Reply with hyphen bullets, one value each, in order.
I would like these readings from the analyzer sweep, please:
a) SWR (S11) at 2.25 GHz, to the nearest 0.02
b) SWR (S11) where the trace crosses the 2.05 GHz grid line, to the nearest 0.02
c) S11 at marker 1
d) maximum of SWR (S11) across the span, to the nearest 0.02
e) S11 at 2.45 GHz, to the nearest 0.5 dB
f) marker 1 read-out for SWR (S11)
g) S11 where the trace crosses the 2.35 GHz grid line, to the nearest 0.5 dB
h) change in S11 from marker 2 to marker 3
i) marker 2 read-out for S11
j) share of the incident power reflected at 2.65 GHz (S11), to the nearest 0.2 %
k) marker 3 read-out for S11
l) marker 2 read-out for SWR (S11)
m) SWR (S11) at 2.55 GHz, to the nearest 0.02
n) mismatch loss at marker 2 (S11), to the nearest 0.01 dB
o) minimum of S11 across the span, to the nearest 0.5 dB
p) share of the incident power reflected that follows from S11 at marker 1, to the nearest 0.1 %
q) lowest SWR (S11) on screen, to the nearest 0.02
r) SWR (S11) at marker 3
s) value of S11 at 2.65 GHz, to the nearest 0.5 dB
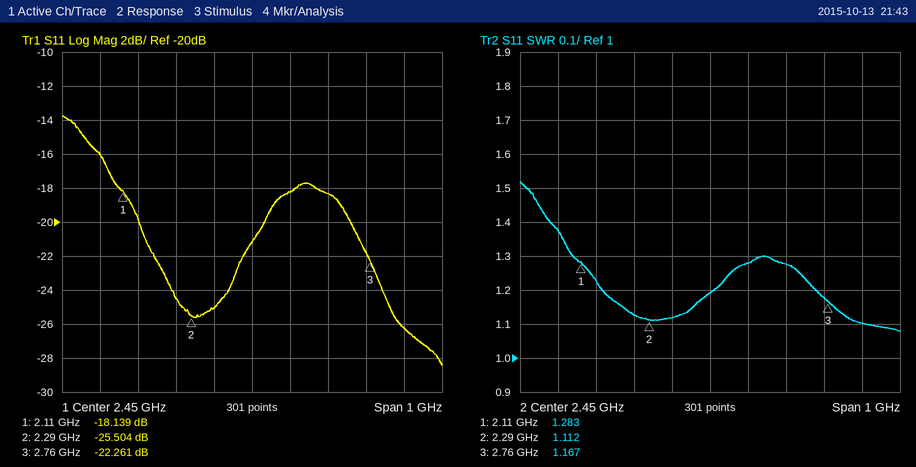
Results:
- 1.12
- 1.38
- -18.139 dB
- 1.52
- -21.0 dB
- 1.283
- -25.0 dB
- 3.243 dB
- -25.504 dB
- 1.4 %
- -22.261 dB
- 1.112
- 1.28
- 0.01 dB
- -28.5 dB
- 1.5 %
- 1.08
- 1.167
- -18.5 dB
